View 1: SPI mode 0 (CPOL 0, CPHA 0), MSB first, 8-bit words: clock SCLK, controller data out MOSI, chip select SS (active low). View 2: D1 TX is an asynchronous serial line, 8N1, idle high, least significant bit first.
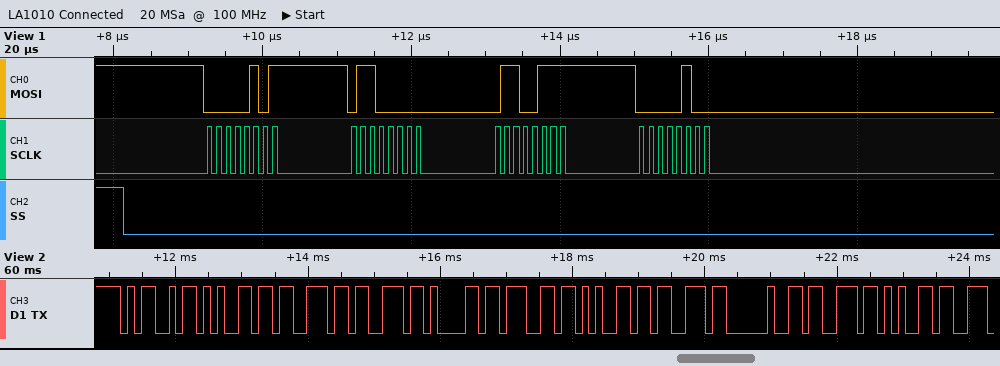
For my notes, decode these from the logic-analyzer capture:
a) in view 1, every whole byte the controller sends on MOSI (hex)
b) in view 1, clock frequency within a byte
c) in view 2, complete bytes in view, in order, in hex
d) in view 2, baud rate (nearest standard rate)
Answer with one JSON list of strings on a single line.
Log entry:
["05 60 67 04", "8 MHz", "0x4D 0x65 0x73 0x73 0x61 0x67 0x65 0x73 0x20 0x73 0x65", "9600 baud"]
